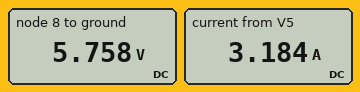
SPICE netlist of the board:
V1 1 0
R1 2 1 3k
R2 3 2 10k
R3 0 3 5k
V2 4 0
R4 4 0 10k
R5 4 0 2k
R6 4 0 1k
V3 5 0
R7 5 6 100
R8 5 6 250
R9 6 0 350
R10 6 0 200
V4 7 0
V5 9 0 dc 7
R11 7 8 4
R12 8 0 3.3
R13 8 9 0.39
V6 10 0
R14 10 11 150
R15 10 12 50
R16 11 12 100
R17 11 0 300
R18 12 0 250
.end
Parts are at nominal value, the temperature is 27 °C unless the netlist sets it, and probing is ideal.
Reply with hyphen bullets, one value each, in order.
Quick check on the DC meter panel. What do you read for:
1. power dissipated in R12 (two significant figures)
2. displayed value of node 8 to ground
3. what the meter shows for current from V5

- 10 W
- 5.758 V
- 3.184 A
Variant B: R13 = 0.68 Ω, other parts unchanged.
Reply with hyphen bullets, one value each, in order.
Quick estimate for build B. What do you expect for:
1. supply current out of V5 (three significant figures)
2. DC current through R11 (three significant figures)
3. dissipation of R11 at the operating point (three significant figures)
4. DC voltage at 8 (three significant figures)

- 2.81 A
- 1.27 A
- 6.47 W
- 5.09 V
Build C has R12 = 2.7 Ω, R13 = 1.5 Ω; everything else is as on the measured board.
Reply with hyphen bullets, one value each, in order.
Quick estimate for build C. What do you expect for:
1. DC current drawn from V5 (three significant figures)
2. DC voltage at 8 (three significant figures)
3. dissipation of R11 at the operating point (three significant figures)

- 2.25 A
- 3.63 V
- 3.29 W
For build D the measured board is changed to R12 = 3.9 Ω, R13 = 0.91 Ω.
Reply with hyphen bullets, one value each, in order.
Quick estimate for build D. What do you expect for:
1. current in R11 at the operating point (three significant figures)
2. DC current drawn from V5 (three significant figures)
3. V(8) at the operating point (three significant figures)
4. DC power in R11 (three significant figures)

- 1.20 A
- 2.43 A
- 4.79 V
- 5.74 W
